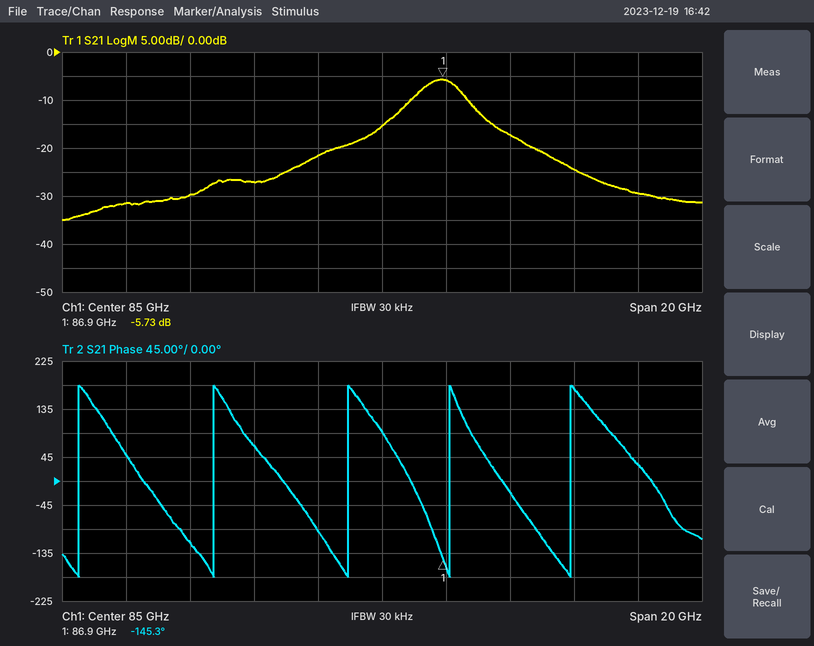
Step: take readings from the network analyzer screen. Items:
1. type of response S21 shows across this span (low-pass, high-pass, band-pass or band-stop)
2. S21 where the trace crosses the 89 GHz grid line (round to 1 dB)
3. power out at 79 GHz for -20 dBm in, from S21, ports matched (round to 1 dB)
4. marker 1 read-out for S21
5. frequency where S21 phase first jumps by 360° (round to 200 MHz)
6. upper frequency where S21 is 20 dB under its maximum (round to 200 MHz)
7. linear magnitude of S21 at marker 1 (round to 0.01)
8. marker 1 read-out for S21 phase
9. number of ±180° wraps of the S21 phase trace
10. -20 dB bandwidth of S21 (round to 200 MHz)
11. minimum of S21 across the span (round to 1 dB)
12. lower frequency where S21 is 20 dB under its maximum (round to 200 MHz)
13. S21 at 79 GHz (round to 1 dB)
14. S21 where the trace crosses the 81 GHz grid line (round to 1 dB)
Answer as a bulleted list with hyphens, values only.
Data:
- band-pass
- -17 dB
- -50 dBm
- -5.73 dB
- 75.6 GHz
- 91.4 GHz
- 0.52
- -145.3°
- 5
- 9.6 GHz
- -35 dB
- 81.8 GHz
- -30 dB
- -27 dB
